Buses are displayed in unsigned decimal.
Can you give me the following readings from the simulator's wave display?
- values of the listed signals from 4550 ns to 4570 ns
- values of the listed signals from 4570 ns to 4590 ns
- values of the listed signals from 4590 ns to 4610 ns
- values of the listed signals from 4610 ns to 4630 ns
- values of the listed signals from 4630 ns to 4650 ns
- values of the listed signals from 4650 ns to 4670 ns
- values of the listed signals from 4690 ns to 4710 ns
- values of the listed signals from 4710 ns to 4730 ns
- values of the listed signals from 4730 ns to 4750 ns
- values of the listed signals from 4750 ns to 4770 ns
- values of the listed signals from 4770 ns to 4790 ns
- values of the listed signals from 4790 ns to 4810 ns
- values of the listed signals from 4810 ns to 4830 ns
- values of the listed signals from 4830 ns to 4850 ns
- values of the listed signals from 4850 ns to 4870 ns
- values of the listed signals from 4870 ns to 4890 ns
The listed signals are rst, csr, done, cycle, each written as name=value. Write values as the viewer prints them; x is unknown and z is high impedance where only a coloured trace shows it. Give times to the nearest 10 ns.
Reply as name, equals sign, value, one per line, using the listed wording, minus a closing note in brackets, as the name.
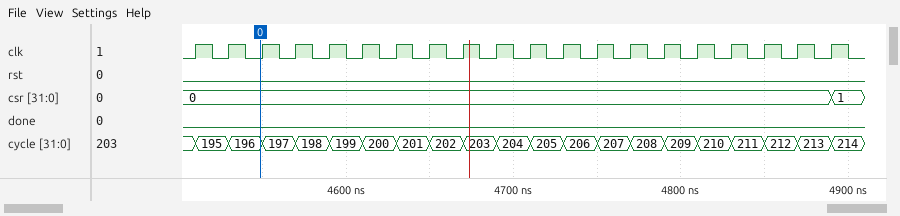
values of the listed signals from 4550 ns to 4570 ns = rst=0, csr=0, done=0, cycle=197
values of the listed signals from 4570 ns to 4590 ns = rst=0, csr=0, done=0, cycle=198
values of the listed signals from 4590 ns to 4610 ns = rst=0, csr=0, done=0, cycle=199
values of the listed signals from 4610 ns to 4630 ns = rst=0, csr=0, done=0, cycle=200
values of the listed signals from 4630 ns to 4650 ns = rst=0, csr=0, done=0, cycle=201
values of the listed signals from 4650 ns to 4670 ns = rst=0, csr=0, done=0, cycle=202
values of the listed signals from 4690 ns to 4710 ns = rst=0, csr=0, done=0, cycle=204
values of the listed signals from 4710 ns to 4730 ns = rst=0, csr=0, done=0, cycle=205
values of the listed signals from 4730 ns to 4750 ns = rst=0, csr=0, done=0, cycle=206
values of the listed signals from 4750 ns to 4770 ns = rst=0, csr=0, done=0, cycle=207
values of the listed signals from 4770 ns to 4790 ns = rst=0, csr=0, done=0, cycle=208
values of the listed signals from 4790 ns to 4810 ns = rst=0, csr=0, done=0, cycle=209
values of the listed signals from 4810 ns to 4830 ns = rst=0, csr=0, done=0, cycle=210
values of the listed signals from 4830 ns to 4850 ns = rst=0, csr=0, done=0, cycle=211
values of the listed signals from 4850 ns to 4870 ns = rst=0, csr=0, done=0, cycle=212
values of the listed signals from 4870 ns to 4890 ns = rst=0, csr=0, done=0, cycle=213
